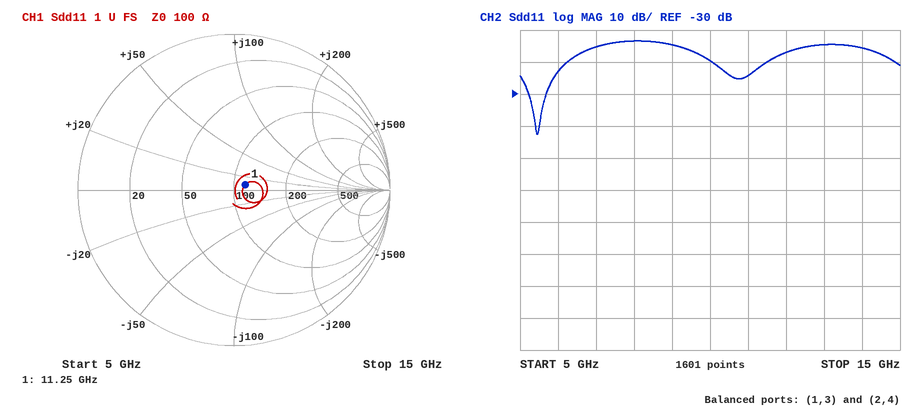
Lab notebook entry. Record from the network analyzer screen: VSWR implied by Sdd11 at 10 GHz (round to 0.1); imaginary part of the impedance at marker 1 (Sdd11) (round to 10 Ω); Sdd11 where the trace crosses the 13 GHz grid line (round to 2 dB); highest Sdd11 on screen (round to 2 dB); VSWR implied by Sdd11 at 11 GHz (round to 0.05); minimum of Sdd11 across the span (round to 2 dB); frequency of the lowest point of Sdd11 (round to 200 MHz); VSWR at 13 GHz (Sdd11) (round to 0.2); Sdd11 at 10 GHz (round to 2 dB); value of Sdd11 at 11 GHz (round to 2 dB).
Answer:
1.2
+10 Ω
-14 dB
-14 dB
1.15
-42 dB
5.4 GHz
1.4
-20 dB
-24 dB
